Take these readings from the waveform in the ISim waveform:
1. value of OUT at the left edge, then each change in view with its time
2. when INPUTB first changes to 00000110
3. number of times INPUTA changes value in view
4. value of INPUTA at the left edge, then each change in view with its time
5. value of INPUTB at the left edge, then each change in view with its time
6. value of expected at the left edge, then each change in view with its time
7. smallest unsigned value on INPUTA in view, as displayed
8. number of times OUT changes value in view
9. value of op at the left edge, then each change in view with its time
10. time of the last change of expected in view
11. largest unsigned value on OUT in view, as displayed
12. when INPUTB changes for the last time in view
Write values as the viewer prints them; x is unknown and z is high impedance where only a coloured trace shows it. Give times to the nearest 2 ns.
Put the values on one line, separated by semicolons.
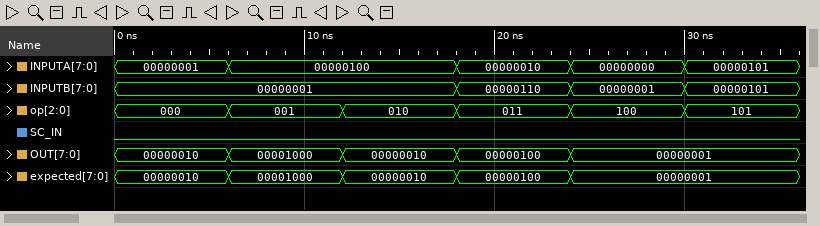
00000010, 00001000 at 6 ns, 00000010 at 12 ns, 00000100 at 18 ns, 00000001 at 24 ns; 18 ns; 4; 00000001, 00000100 at 6 ns, 00000010 at 18 ns, 00000000 at 24 ns, 00000101 at 30 ns; 00000001, 00000110 at 18 ns, 00000001 at 24 ns, 00000101 at 30 ns; 00000010, 00001000 at 6 ns, 00000010 at 12 ns, 00000100 at 18 ns, 00000001 at 24 ns; 00000000; 4; 000, 001 at 6 ns, 010 at 12 ns, 011 at 18 ns, 100 at 24 ns, 101 at 30 ns; 24 ns; 00001000; 30 ns
